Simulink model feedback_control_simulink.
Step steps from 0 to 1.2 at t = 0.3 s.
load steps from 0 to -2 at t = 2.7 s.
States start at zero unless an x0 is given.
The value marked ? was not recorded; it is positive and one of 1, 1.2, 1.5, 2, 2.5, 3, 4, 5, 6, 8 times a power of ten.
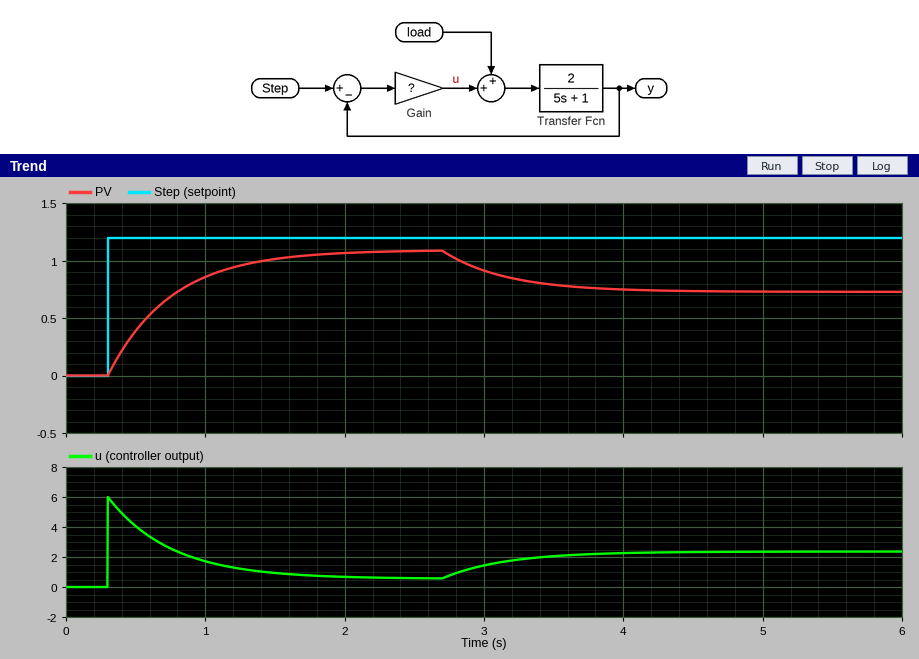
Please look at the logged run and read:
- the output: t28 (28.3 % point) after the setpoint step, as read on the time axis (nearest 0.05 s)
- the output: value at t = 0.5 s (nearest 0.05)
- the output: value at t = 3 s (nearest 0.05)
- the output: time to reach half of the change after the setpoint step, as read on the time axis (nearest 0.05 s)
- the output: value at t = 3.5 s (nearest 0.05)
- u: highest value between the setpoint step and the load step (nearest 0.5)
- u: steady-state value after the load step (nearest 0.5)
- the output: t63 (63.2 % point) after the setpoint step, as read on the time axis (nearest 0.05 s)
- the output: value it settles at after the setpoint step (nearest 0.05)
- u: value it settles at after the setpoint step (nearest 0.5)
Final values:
0.45 s
0.40
0.90
0.60 s
0.80
6.0
2.5
0.75 s
1.10
0.5
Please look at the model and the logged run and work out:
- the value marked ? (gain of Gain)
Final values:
5
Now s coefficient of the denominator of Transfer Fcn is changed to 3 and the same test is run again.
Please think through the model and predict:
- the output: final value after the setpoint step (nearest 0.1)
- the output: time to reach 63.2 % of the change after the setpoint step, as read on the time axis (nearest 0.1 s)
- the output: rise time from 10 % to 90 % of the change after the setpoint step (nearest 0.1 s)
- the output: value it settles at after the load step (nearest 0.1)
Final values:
1.1
0.6 s
0.6 s
0.7
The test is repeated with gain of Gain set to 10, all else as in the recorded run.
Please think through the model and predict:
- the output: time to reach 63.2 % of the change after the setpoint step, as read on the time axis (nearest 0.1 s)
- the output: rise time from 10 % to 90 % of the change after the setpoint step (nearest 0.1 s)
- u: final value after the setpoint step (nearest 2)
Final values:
0.5 s
0.5 s
0
